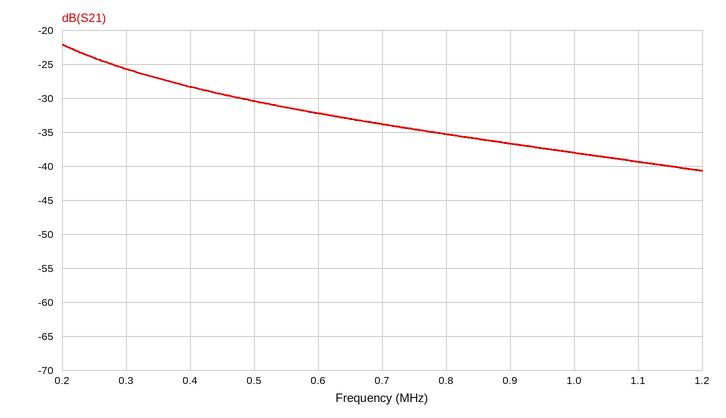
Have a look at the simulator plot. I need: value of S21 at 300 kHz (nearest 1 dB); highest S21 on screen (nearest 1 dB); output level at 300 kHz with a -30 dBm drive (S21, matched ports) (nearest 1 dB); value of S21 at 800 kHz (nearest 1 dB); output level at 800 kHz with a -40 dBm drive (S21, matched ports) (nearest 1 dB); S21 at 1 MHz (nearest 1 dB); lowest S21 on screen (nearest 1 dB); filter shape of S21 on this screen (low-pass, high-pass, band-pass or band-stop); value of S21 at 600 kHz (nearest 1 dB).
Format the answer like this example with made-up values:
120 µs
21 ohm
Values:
-26 dB
-22 dB
-56 dBm
-35 dB
-75 dBm
-38 dB
-41 dB
low-pass
-32 dB
